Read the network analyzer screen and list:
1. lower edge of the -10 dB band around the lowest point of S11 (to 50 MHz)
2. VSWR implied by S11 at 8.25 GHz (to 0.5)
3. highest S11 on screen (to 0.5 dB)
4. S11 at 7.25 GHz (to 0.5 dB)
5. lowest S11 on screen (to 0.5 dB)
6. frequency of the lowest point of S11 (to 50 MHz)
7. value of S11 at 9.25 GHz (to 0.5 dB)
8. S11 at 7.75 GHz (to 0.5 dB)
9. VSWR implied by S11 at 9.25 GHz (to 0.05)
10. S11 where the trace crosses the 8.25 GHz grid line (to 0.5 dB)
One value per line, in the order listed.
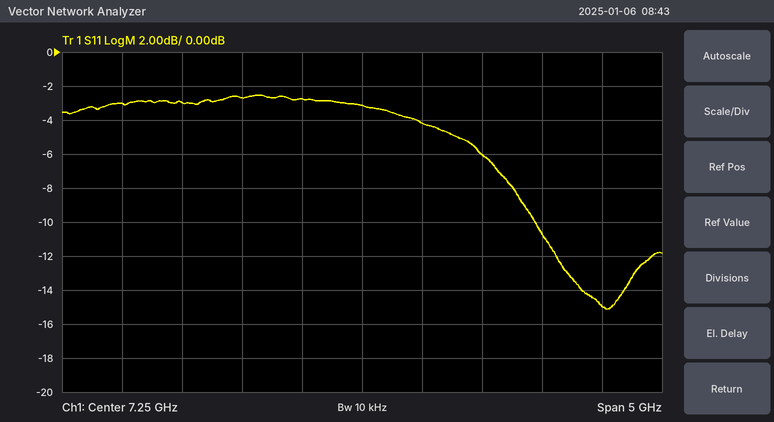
8.70 GHz
3.0
-2.5 dB
-3.0 dB
-15.0 dB
9.30 GHz
-15.0 dB
-4.0 dB
1.45
-6.0 dB
